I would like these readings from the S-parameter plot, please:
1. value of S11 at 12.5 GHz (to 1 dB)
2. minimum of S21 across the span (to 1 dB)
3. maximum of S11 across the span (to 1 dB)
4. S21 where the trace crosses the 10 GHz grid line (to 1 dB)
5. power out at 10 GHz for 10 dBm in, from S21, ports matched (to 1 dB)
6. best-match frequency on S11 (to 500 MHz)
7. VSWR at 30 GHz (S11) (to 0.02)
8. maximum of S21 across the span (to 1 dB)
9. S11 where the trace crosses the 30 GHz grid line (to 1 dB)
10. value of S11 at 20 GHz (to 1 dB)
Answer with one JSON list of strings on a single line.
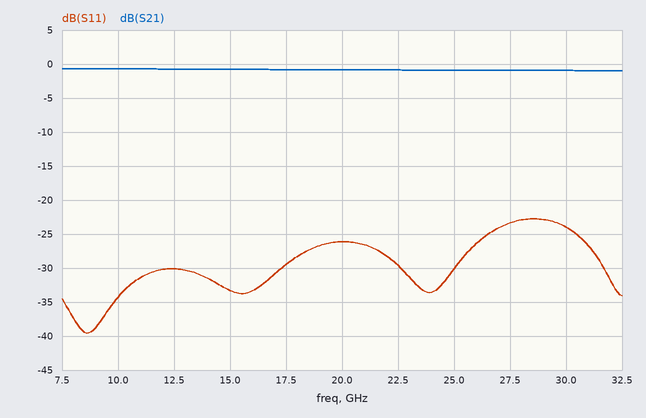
["-30 dB", "-1 dB", "-23 dB", "-1 dB", "9 dBm", "8.5 GHz", "1.14", "-1 dB", "-24 dB", "-26 dB"]
